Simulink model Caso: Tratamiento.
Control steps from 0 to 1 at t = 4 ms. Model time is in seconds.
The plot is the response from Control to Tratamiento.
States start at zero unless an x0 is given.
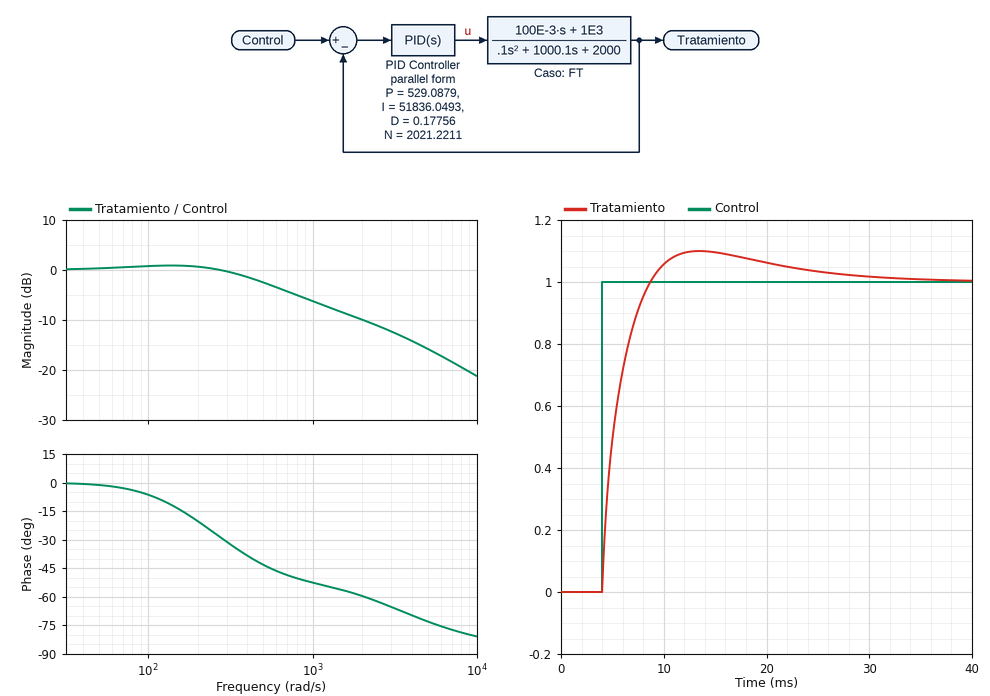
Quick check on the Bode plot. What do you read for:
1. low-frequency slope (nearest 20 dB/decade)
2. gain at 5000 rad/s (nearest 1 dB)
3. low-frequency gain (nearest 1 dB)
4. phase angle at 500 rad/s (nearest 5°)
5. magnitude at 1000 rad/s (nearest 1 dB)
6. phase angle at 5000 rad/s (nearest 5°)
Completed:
0 dB/decade
-16 dB
0 dB
-45°
-6 dB
-75°
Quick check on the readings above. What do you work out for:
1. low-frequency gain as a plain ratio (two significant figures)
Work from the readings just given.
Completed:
1.0
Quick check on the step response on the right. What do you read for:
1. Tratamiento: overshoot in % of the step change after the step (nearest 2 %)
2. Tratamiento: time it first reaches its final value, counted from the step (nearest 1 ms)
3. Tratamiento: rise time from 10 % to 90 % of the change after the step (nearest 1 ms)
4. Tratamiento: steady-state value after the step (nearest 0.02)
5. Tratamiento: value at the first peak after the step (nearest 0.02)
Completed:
10 %
5 ms
3 ms
1.00
1.10
